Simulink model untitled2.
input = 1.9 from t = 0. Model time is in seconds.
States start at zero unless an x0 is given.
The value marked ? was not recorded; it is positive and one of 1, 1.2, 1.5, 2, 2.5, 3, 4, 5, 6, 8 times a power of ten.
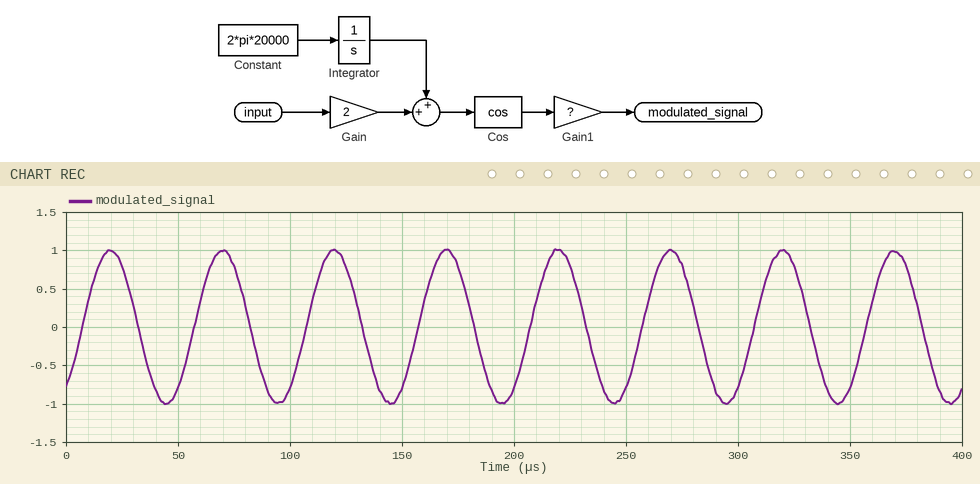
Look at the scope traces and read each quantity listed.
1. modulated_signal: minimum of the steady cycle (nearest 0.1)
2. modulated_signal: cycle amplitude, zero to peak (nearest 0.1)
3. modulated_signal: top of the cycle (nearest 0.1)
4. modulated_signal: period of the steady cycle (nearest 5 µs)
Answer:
-1.0
1.0
1.0
50 µs
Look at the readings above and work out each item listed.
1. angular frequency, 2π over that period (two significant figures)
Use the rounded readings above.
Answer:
0.13 rad/µs
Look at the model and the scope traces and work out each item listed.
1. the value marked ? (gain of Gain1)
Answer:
1
